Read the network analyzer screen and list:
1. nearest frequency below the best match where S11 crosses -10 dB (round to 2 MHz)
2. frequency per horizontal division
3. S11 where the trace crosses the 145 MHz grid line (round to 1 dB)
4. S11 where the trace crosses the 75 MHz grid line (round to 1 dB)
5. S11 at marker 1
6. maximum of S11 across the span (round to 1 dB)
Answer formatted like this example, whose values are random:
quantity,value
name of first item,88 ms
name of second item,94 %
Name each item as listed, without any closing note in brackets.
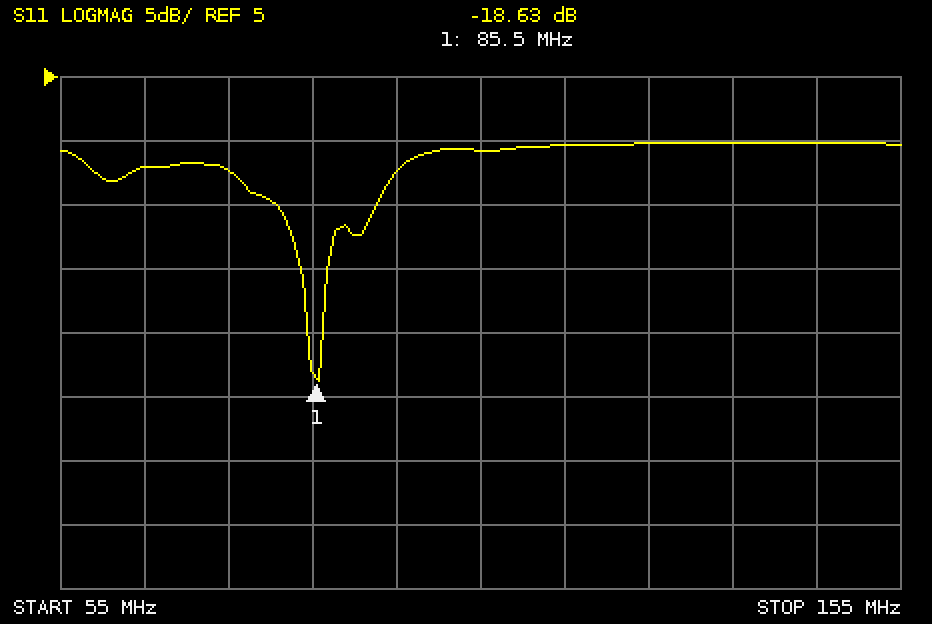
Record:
quantity,value
nearest frequency below the best match where S11 crosses -10 dB,84 MHz
frequency per horizontal division,10 MHz
S11 where the trace crosses the 145 MHz grid line,0 dB
S11 where the trace crosses the 75 MHz grid line,-2 dB
S11 at marker 1,-18.63 dB
maximum of S11 across the span,0 dB
